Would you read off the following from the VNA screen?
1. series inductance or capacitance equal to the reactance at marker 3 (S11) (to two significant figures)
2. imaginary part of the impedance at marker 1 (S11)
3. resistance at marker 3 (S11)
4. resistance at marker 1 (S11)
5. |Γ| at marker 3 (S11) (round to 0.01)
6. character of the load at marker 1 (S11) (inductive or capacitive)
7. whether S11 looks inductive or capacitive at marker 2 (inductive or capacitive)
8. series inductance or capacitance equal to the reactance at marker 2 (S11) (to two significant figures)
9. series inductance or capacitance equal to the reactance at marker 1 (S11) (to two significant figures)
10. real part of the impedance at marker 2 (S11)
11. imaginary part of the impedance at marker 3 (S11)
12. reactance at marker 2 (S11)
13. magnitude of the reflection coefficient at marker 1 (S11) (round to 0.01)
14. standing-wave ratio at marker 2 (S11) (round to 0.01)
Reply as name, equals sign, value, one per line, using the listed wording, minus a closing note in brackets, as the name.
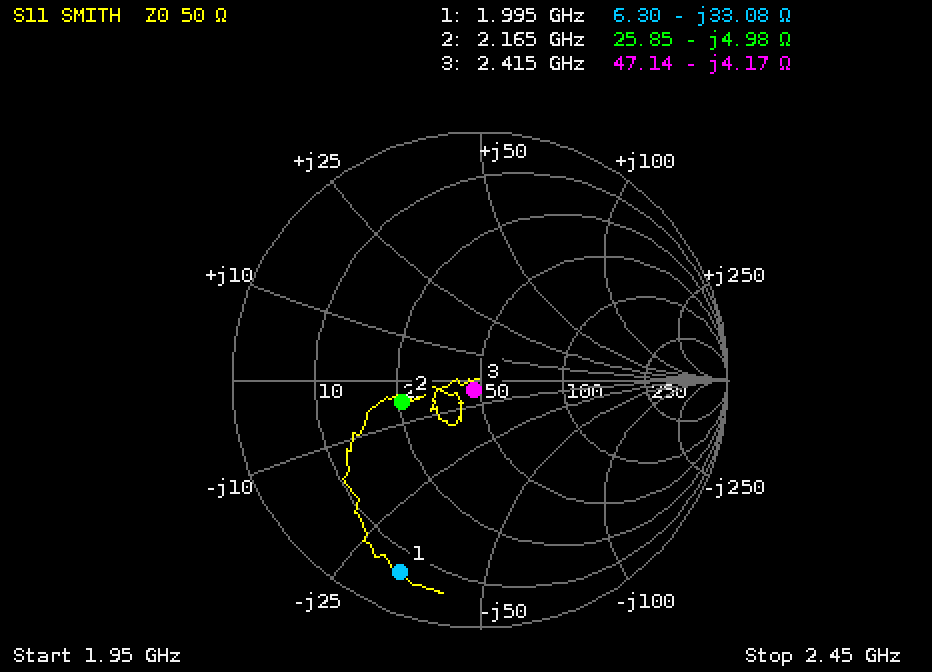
series inductance or capacitance equal to the reactance at marker 3 (S11) = 16 pF
imaginary part of the impedance at marker 1 = -33.08 Ω
resistance at marker 3 = 47.14 Ω
resistance at marker 1 = 6.30 Ω
|Γ| at marker 3 (S11) = 0.05
character of the load at marker 1 (S11) = capacitive
whether S11 looks inductive or capacitive at marker 2 = capacitive
series inductance or capacitance equal to the reactance at marker 2 (S11) = 15 pF
series inductance or capacitance equal to the reactance at marker 1 (S11) = 2.4 pF
real part of the impedance at marker 2 = 25.85 Ω
imaginary part of the impedance at marker 3 = -4.17 Ω
reactance at marker 2 = -4.98 Ω
magnitude of the reflection coefficient at marker 1 (S11) = 0.84
standing-wave ratio at marker 2 (S11) = 1.96
